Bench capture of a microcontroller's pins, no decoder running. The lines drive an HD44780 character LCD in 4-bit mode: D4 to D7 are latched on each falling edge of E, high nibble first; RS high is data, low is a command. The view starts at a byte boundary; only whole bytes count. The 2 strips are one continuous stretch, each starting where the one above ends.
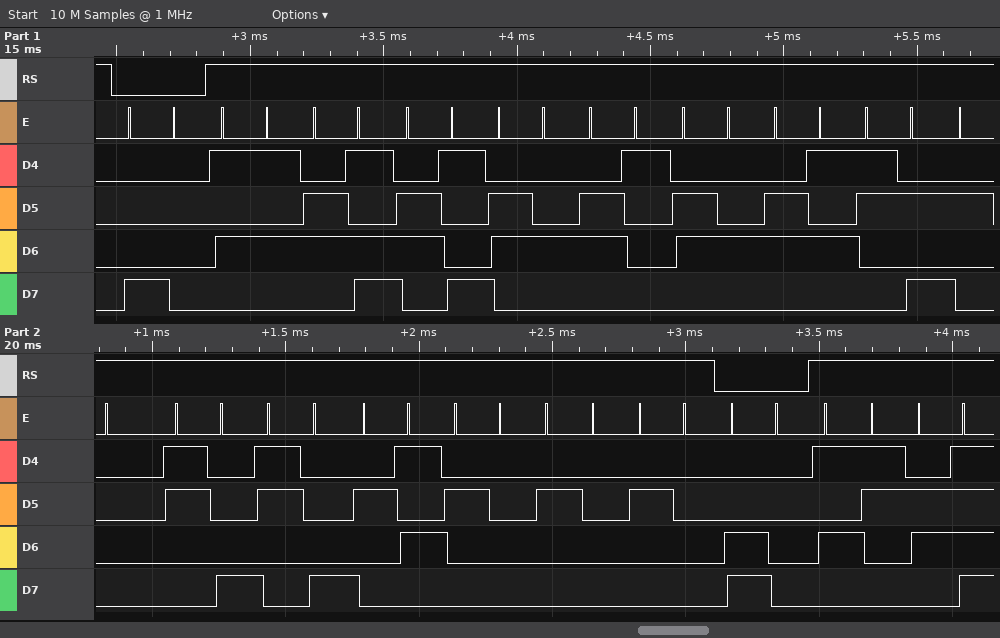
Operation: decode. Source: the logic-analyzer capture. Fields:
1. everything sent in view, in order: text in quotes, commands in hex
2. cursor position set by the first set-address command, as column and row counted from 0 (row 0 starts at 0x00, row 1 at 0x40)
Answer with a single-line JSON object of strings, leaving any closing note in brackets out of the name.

{"everything sent in view, in order: text in quotes, commands in hex": "0x80 \"Umidade: 88%   \" 0xC0 \"So\"", "cursor position set by the first set-address command, as column and row counted from 0": "column 0, row 0"}
